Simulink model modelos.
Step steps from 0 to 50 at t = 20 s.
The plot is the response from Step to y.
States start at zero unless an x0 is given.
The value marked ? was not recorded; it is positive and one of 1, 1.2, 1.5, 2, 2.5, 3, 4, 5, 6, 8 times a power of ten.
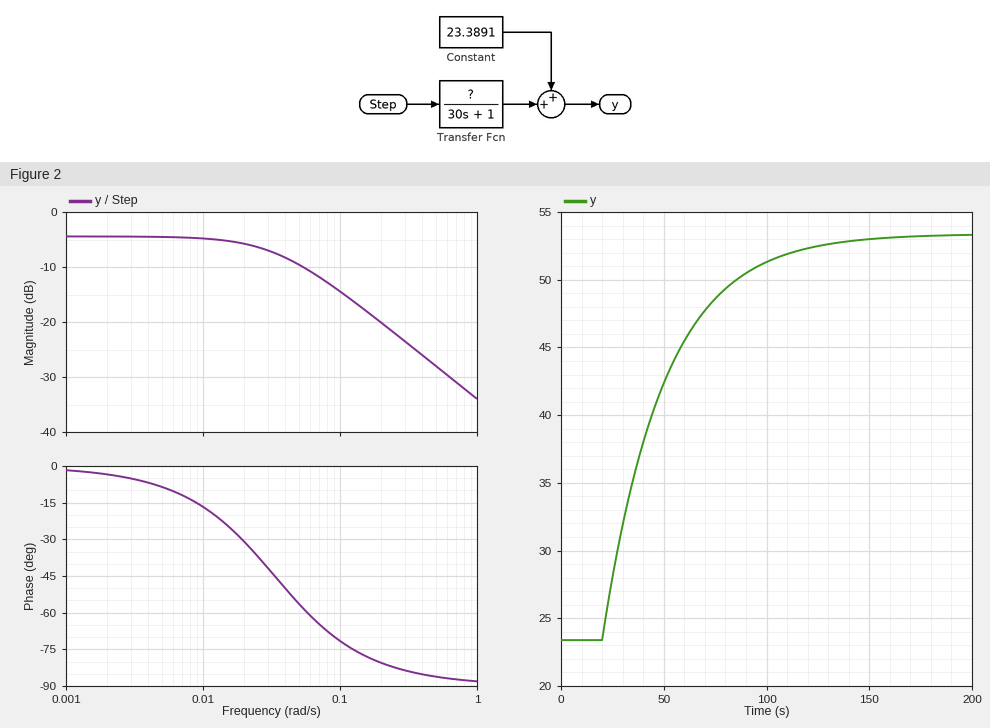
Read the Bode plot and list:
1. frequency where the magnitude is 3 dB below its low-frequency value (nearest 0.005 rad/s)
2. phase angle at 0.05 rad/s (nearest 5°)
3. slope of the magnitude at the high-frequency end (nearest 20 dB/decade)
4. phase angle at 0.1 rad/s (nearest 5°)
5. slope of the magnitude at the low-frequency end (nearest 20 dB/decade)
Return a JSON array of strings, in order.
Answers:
["0.035 rad/s", "-55°", "-20 dB/decade", "-70°", "0 dB/decade"]
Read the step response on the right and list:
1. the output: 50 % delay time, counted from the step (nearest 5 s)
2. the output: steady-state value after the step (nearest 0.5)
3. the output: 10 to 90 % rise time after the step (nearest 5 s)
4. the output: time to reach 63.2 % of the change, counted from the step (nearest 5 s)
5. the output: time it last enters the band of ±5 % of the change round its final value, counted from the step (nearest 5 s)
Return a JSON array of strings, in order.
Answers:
["20 s", "53.5", "65 s", "30 s", "90 s"]
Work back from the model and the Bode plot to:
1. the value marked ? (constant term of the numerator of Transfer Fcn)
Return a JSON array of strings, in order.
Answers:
["0.6"]
